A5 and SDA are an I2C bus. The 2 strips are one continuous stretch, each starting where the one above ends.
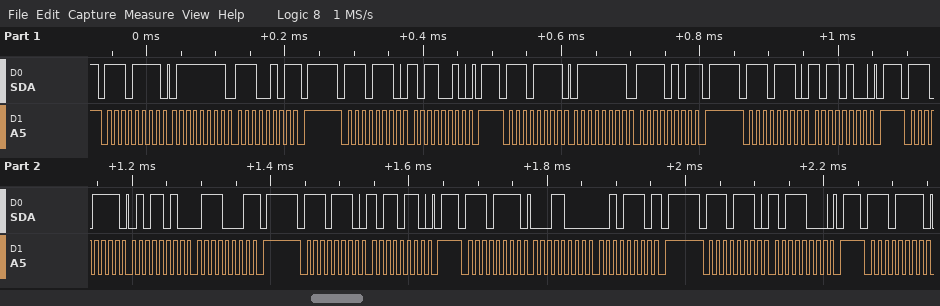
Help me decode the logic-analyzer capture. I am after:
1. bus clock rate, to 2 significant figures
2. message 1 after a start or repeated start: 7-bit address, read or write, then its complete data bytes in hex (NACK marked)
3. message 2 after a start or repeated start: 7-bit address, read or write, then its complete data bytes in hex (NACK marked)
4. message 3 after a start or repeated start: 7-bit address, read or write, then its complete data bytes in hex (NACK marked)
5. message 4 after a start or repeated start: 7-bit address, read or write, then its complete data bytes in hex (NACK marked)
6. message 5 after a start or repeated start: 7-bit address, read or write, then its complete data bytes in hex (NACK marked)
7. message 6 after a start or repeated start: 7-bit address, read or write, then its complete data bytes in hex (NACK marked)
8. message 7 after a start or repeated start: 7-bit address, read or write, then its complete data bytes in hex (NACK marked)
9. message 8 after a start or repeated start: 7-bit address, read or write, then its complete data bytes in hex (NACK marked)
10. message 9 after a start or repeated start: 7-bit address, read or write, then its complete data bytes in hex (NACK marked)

100 kHz
0x77 read: 7F E5 NACK
0x77 write: B2
0x77 read: 7F F5 NACK
0x77 write: B4
0x77 read: 5A 71 NACK
0x77 write: B6
0x77 read: 18 2E NACK
0x77 write: B8
0x77 read
